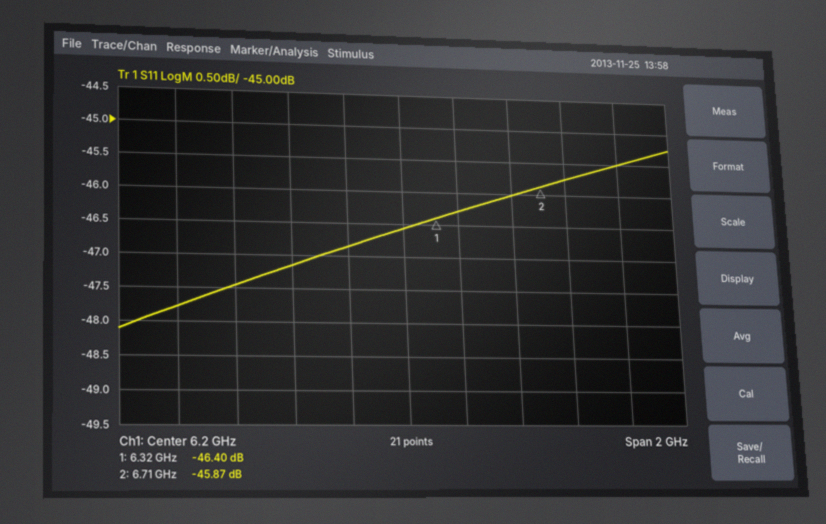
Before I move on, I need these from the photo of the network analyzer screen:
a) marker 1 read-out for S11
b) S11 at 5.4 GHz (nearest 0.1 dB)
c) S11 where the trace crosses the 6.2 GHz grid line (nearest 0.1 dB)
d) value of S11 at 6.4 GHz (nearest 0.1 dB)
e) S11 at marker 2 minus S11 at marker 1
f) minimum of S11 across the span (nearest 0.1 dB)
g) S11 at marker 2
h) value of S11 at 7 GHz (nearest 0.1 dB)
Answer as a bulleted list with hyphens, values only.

- -46.40 dB
- -47.8 dB
- -46.6 dB
- -46.3 dB
- 0.53 dB
- -48.1 dB
- -45.87 dB
- -45.5 dB
